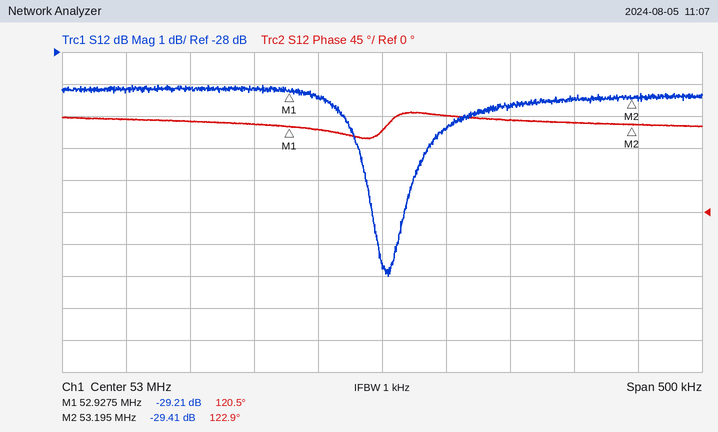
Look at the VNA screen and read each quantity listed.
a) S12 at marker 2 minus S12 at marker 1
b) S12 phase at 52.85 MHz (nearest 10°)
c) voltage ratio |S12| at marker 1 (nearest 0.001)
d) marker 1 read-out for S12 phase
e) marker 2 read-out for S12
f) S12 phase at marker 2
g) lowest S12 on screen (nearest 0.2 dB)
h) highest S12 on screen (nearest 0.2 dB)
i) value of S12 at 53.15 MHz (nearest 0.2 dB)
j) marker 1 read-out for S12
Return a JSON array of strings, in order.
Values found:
["-0.20 dB", "130°", "0.035", "120.5°", "-29.41 dB", "122.9°", "-35.0 dB", "-29.0 dB", "-29.4 dB", "-29.21 dB"]
